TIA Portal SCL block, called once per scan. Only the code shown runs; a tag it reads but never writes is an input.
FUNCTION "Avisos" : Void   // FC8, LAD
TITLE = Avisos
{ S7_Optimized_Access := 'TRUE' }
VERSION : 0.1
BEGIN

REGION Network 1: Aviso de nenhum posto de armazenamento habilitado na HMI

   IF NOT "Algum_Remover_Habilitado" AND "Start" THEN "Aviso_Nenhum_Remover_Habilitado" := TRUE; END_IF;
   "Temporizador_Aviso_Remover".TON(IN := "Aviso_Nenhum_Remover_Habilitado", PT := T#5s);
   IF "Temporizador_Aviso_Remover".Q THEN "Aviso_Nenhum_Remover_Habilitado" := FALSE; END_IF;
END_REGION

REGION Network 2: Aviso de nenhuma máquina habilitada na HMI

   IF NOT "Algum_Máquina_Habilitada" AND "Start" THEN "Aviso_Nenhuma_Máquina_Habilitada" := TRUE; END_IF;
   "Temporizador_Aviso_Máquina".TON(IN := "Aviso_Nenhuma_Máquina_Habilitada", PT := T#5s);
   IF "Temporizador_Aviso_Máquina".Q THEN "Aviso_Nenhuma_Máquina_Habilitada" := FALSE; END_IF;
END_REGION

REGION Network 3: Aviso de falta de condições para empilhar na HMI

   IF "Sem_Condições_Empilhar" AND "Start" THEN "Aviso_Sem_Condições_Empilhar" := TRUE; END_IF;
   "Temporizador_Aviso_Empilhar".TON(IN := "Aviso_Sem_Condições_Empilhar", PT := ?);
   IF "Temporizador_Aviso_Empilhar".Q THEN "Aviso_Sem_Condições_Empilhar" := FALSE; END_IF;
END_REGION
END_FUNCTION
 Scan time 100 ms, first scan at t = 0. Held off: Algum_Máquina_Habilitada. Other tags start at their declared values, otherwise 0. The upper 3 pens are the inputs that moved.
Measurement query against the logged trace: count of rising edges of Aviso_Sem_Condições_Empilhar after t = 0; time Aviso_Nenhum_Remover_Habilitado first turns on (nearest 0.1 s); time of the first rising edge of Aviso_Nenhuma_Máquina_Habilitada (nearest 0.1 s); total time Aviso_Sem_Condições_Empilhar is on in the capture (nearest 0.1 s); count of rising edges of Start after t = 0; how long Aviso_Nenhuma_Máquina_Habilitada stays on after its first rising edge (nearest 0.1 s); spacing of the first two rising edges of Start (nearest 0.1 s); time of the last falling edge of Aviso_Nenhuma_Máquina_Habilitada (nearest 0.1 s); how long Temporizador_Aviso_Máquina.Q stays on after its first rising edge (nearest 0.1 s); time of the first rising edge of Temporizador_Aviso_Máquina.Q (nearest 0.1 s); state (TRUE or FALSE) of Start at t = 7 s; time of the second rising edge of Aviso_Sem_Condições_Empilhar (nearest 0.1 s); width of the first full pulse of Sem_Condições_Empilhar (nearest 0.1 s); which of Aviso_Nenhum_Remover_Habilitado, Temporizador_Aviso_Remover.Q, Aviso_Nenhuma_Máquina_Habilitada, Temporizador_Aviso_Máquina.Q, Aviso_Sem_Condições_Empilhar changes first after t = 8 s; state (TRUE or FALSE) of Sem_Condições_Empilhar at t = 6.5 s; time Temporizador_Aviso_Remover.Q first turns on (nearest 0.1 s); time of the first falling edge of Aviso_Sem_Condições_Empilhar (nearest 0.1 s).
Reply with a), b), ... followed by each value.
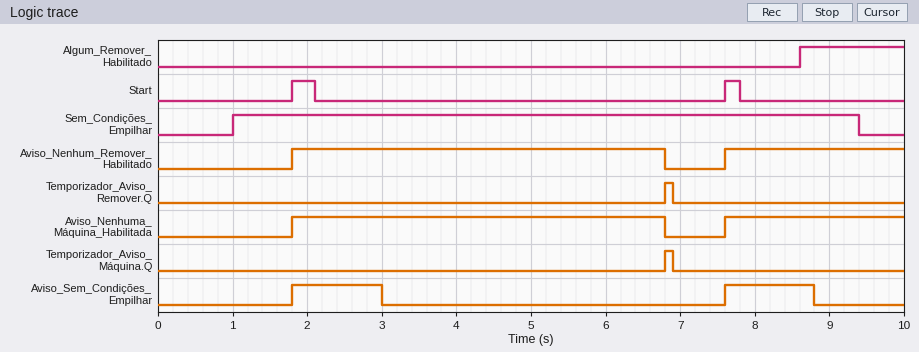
a) 2
b) 1.8 s
c) 1.8 s
d) 2.4 s
e) 2
f) 5.0 s
g) 5.8 s
h) 6.8 s
i) 0.1 s
j) 6.8 s
k) FALSE
l) 7.6 s
m) 8.4 s
n) Aviso_Sem_Condições_Empilhar
o) TRUE
p) 6.8 s
q) 3.0 s
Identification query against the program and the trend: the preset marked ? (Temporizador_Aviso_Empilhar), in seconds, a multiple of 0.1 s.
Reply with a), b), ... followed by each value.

a) 1.2 s
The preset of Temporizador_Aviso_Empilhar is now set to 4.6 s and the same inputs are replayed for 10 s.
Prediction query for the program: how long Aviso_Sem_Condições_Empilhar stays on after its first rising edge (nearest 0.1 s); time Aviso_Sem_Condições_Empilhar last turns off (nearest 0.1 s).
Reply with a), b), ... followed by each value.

a) 4.6 s
b) 6.4 s
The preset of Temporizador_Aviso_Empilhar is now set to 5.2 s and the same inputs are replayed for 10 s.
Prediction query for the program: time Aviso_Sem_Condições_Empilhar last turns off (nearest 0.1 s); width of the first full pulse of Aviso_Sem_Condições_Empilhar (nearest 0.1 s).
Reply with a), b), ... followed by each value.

a) 7.0 s
b) 5.2 s
